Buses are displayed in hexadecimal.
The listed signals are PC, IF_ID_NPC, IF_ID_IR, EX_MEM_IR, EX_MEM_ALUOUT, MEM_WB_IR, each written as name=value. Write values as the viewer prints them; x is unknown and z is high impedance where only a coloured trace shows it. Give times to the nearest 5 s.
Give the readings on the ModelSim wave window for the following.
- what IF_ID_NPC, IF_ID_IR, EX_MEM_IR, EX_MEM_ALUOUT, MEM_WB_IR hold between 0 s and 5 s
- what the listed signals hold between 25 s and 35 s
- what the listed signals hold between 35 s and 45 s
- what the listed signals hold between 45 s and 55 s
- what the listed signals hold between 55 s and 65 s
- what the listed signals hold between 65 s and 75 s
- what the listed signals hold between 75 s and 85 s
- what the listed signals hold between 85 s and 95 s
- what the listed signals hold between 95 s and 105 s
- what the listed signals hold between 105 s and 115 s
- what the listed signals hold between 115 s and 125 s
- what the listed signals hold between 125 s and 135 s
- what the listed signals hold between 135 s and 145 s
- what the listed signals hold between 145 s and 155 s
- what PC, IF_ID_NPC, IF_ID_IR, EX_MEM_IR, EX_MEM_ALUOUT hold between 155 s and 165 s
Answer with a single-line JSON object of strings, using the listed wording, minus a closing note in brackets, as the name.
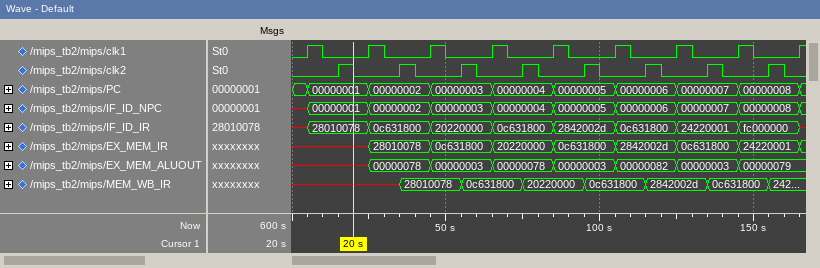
{"what IF_ID_NPC, IF_ID_IR, EX_MEM_IR, EX_MEM_ALUOUT, MEM_WB_IR hold between 0 s and 5 s": "IF_ID_NPC=x, IF_ID_IR=x, EX_MEM_IR=x, EX_MEM_ALUOUT=x, MEM_WB_IR=x", "what the listed signals hold between 25 s and 35 s": "PC=00000002, IF_ID_NPC=00000002, IF_ID_IR=0c631800, EX_MEM_IR=28010078, EX_MEM_ALUOUT=00000078, MEM_WB_IR=x", "what the listed signals hold between 35 s and 45 s": "PC=00000002, IF_ID_NPC=00000002, IF_ID_IR=0c631800, EX_MEM_IR=28010078, EX_MEM_ALUOUT=00000078, MEM_WB_IR=28010078", "what the listed signals hold between 45 s and 55 s": "PC=00000003, IF_ID_NPC=00000003, IF_ID_IR=20220000, EX_MEM_IR=0c631800, EX_MEM_ALUOUT=00000003, MEM_WB_IR=28010078", "what the listed signals hold between 55 s and 65 s": "PC=00000003, IF_ID_NPC=00000003, IF_ID_IR=20220000, EX_MEM_IR=0c631800, EX_MEM_ALUOUT=00000003, MEM_WB_IR=0c631800", "what the listed signals hold between 65 s and 75 s": "PC=00000004, IF_ID_NPC=00000004, IF_ID_IR=0c631800, EX_MEM_IR=20220000, EX_MEM_ALUOUT=00000078, MEM_WB_IR=0c631800", "what the listed signals hold between 75 s and 85 s": "PC=00000004, IF_ID_NPC=00000004, IF_ID_IR=0c631800, EX_MEM_IR=20220000, EX_MEM_ALUOUT=00000078, MEM_WB_IR=20220000", "what the listed signals hold between 85 s and 95 s": "PC=00000005, IF_ID_NPC=00000005, IF_ID_IR=2842002d, EX_MEM_IR=0c631800, EX_MEM_ALUOUT=00000003, MEM_WB_IR=20220000", "what the listed signals hold between 95 s and 105 s": "PC=00000005, IF_ID_NPC=00000005, IF_ID_IR=2842002d, EX_MEM_IR=0c631800, EX_MEM_ALUOUT=00000003, MEM_WB_IR=0c631800", "what the listed signals hold between 105 s and 115 s": "PC=00000006, IF_ID_NPC=00000006, IF_ID_IR=0c631800, EX_MEM_IR=2842002d, EX_MEM_ALUOUT=00000082, MEM_WB_IR=0c631800", "what the listed signals hold between 115 s and 125 s": "PC=00000006, IF_ID_NPC=00000006, IF_ID_IR=0c631800, EX_MEM_IR=2842002d, EX_MEM_ALUOUT=00000082, MEM_WB_IR=2842002d", "what the listed signals hold between 125 s and 135 s": "PC=00000007, IF_ID_NPC=00000007, IF_ID_IR=24220001, EX_MEM_IR=0c631800, EX_MEM_ALUOUT=00000003, MEM_WB_IR=2842002d", "what the listed signals hold between 135 s and 145 s": "PC=00000007, IF_ID_NPC=00000007, IF_ID_IR=24220001, EX_MEM_IR=0c631800, EX_MEM_ALUOUT=00000003, MEM_WB_IR=0c631800", "what the listed signals hold between 145 s and 155 s": "PC=00000008, IF_ID_NPC=00000008, IF_ID_IR=fc000000, EX_MEM_IR=24220001, EX_MEM_ALUOUT=00000079, MEM_WB_IR=0c631800", "what PC, IF_ID_NPC, IF_ID_IR, EX_MEM_IR, EX_MEM_ALUOUT hold between 155 s and 165 s": "PC=00000008, IF_ID_NPC=00000008, IF_ID_IR=fc000000, EX_MEM_IR=24220001, EX_MEM_ALUOUT=00000079"}
